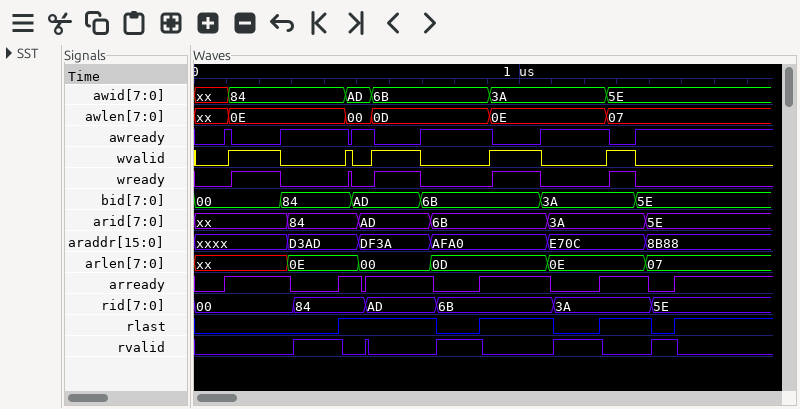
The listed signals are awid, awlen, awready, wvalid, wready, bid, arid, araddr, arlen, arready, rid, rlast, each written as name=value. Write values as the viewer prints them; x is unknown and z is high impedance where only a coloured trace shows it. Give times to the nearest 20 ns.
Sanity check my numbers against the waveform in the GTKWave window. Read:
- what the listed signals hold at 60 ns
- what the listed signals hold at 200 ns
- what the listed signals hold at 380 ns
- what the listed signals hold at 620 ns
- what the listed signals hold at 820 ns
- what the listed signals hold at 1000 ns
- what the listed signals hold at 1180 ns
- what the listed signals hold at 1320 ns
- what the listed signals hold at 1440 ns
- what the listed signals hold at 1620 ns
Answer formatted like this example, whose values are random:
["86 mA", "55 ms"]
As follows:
["awid=xx, awlen=xx, awready=0, wvalid=0, wready=0, bid=00, arid=xx, araddr=xxxx, arlen=xx, arready=0, rid=00, rlast=0", "awid=84, awlen=0E, awready=0, wvalid=1, wready=1, bid=00, arid=xx, araddr=xxxx, arlen=xx, arready=1, rid=00, rlast=0", "awid=84, awlen=0E, awready=1, wvalid=0, wready=0, bid=84, arid=84, araddr=D3AD, arlen=0E, arready=0, rid=84, rlast=0", "awid=6B, awlen=0D, awready=0, wvalid=1, wready=1, bid=AD, arid=AD, araddr=DF3A, arlen=00, arready=1, rid=AD, rlast=1", "awid=6B, awlen=0D, awready=1, wvalid=0, wready=0, bid=6B, arid=6B, araddr=AFA0, arlen=0D, arready=0, rid=6B, rlast=0", "awid=3A, awlen=0E, awready=0, wvalid=1, wready=1, bid=6B, arid=6B, araddr=AFA0, arlen=0D, arready=1, rid=6B, rlast=1", "awid=3A, awlen=0E, awready=1, wvalid=0, wready=0, bid=3A, arid=3A, araddr=E70C, arlen=0E, arready=0, rid=3A, rlast=0", "awid=5E, awlen=07, awready=0, wvalid=1, wready=1, bid=3A, arid=3A, araddr=E70C, arlen=0E, arready=1, rid=3A, rlast=1", "awid=5E, awlen=07, awready=1, wvalid=0, wready=0, bid=5E, arid=5E, araddr=8B88, arlen=07, arready=0, rid=5E, rlast=0", "awid=5E, awlen=07, awready=1, wvalid=0, wready=0, bid=5E, arid=5E, araddr=8B88, arlen=07, arready=1, rid=5E, rlast=1"]
